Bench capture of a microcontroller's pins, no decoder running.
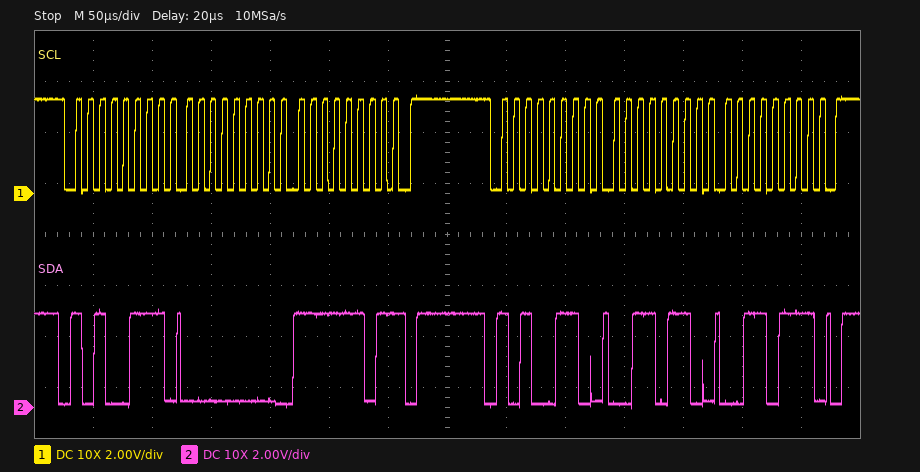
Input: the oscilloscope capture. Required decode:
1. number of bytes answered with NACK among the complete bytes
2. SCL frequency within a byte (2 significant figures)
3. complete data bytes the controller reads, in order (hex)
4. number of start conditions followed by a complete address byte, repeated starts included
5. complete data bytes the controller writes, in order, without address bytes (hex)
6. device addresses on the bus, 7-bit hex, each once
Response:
1
100 kHz
00 FD
2
36 37
0x53
